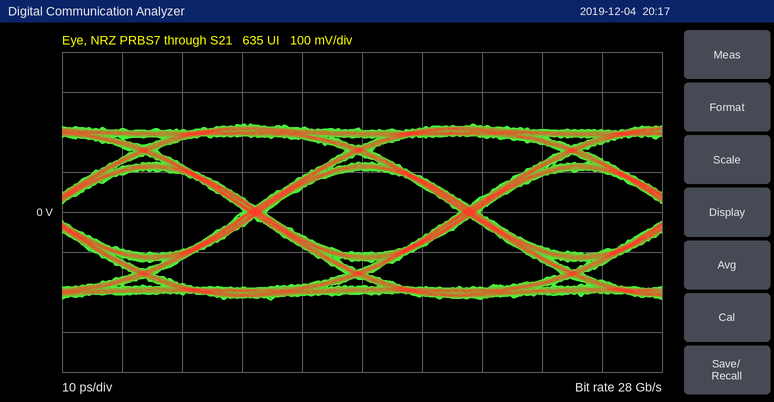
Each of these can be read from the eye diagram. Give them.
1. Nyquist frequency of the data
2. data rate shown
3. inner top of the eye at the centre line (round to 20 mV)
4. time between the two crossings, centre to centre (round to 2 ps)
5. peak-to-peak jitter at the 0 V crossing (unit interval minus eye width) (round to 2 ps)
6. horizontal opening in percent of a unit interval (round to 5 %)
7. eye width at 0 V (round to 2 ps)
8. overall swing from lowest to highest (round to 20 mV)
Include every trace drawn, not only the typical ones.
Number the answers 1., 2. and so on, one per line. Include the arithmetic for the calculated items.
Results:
1. 14 GHz
2. 28 Gb/s
3. 100 mV
4. 36 ps
5. 4 ps
6. 32 ps / 36 ps ≈ 88.9 %, so 90 % to the nearest 5 %
7. 32 ps
8. 440 mV
